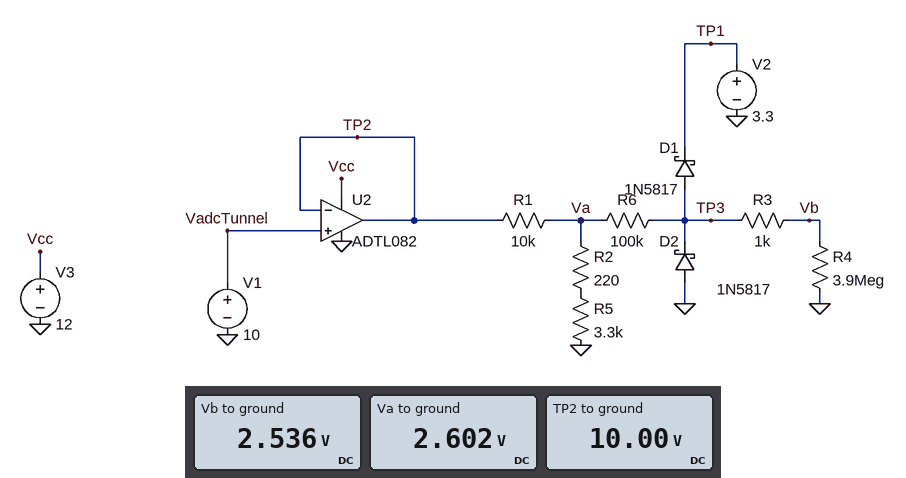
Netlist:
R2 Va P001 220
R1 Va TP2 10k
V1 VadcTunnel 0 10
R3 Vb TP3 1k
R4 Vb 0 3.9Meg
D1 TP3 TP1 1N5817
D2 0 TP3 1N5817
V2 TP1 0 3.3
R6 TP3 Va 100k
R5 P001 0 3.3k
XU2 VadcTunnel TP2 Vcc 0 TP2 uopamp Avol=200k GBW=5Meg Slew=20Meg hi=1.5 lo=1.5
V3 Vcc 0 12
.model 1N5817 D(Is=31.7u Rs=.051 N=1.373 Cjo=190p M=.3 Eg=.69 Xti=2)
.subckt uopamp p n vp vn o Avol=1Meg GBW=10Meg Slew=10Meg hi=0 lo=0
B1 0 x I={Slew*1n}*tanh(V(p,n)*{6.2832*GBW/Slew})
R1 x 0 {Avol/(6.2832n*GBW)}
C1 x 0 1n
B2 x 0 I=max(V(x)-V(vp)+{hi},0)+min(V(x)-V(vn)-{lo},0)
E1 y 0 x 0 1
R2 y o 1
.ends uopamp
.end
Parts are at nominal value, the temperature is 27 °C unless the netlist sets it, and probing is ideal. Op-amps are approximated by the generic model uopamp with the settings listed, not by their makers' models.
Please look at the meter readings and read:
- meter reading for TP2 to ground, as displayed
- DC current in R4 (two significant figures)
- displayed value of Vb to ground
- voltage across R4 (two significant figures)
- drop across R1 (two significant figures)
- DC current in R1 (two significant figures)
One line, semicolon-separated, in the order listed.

10.00 V; 650 nA; 2.536 V; 2.5 V; 7.4 V; 740 µA
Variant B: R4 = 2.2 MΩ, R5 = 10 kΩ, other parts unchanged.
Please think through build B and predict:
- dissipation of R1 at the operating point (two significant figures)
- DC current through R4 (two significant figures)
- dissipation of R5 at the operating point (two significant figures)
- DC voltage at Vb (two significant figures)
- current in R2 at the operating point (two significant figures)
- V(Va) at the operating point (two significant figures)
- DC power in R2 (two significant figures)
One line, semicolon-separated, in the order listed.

2.5 mW; 1.5 µA; 2.4 mW; 3.3 V; 490 µA; 5.0 V; 52 µW
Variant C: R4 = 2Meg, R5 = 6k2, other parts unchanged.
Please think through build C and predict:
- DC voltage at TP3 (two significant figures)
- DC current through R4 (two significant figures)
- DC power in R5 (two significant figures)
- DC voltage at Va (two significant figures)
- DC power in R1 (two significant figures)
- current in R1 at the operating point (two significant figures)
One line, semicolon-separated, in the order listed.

3.2 V; 1.6 µA; 2.3 mW; 3.9 V; 3.7 mW; 610 µA
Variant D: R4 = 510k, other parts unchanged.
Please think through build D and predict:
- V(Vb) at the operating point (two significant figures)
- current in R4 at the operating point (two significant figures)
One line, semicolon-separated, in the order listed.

2.2 V; 4.2 µA
